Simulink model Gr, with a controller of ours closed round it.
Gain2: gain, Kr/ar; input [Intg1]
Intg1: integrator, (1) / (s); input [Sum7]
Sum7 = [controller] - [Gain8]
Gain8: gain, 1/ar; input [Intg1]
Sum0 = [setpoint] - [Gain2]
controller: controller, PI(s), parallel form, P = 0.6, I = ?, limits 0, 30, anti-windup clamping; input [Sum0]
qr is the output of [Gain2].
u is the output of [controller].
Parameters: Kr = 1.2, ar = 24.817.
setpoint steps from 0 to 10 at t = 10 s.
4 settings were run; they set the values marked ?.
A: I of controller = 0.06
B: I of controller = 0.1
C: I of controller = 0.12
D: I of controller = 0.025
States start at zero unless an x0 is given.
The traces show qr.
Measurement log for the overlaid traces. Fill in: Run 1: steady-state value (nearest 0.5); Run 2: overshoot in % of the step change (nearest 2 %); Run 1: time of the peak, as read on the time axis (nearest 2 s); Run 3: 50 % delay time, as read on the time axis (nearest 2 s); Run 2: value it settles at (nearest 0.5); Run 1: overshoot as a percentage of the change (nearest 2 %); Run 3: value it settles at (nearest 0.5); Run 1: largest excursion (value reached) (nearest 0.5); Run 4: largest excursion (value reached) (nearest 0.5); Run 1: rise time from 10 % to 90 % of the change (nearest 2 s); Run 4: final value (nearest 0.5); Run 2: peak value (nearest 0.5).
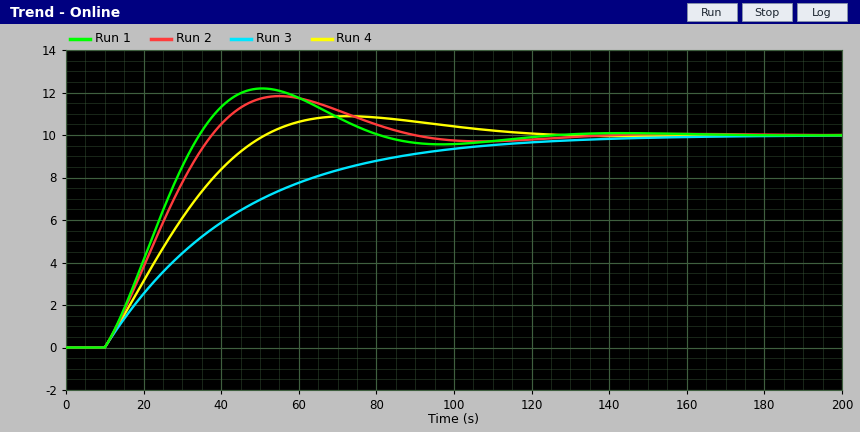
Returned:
10.0
18 %
50 s
34 s
10.0
22 %
10.0
12.0
11.0
18 s
10.0
12.0
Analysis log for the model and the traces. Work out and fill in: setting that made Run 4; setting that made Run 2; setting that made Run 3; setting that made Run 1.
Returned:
A
B
D
C
